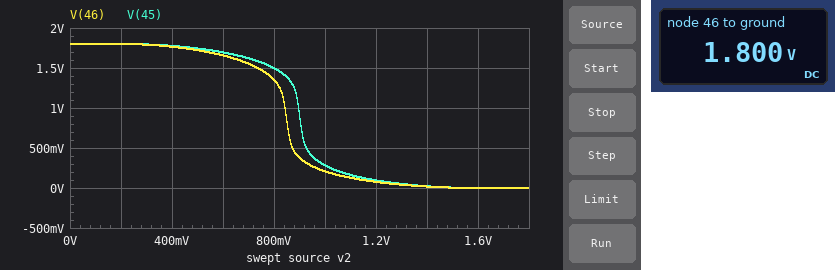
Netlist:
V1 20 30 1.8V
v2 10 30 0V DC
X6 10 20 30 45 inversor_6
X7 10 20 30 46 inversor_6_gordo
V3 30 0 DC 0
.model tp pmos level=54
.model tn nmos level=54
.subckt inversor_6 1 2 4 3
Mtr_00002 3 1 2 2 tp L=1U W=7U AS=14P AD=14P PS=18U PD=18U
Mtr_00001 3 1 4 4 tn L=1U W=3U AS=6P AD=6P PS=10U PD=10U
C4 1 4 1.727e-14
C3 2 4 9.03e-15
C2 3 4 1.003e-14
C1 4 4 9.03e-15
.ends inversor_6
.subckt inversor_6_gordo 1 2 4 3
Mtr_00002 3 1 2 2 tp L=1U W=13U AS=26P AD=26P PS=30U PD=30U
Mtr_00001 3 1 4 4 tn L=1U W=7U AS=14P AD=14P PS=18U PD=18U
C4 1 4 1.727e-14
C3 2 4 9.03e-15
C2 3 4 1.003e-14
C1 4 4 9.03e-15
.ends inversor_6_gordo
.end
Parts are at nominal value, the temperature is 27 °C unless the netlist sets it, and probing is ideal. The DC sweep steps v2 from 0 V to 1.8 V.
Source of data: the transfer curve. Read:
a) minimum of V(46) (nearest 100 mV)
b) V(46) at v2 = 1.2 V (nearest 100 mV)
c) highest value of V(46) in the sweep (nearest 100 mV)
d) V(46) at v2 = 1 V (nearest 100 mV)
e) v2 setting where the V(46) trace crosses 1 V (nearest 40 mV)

0 V
100 mV
1.8 V
200 mV
840 mV
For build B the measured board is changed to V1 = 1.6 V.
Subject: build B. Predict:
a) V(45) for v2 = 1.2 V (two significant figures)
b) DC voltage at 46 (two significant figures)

25 mV
1.6 V
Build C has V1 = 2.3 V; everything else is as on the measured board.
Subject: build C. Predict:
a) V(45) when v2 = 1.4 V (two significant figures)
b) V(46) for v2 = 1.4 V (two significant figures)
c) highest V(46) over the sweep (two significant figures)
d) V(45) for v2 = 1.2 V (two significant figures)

240 mV
190 mV
2.3 V
610 mV
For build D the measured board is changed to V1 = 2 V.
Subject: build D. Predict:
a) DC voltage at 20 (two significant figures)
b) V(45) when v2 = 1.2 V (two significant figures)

2.0 V
210 mV
